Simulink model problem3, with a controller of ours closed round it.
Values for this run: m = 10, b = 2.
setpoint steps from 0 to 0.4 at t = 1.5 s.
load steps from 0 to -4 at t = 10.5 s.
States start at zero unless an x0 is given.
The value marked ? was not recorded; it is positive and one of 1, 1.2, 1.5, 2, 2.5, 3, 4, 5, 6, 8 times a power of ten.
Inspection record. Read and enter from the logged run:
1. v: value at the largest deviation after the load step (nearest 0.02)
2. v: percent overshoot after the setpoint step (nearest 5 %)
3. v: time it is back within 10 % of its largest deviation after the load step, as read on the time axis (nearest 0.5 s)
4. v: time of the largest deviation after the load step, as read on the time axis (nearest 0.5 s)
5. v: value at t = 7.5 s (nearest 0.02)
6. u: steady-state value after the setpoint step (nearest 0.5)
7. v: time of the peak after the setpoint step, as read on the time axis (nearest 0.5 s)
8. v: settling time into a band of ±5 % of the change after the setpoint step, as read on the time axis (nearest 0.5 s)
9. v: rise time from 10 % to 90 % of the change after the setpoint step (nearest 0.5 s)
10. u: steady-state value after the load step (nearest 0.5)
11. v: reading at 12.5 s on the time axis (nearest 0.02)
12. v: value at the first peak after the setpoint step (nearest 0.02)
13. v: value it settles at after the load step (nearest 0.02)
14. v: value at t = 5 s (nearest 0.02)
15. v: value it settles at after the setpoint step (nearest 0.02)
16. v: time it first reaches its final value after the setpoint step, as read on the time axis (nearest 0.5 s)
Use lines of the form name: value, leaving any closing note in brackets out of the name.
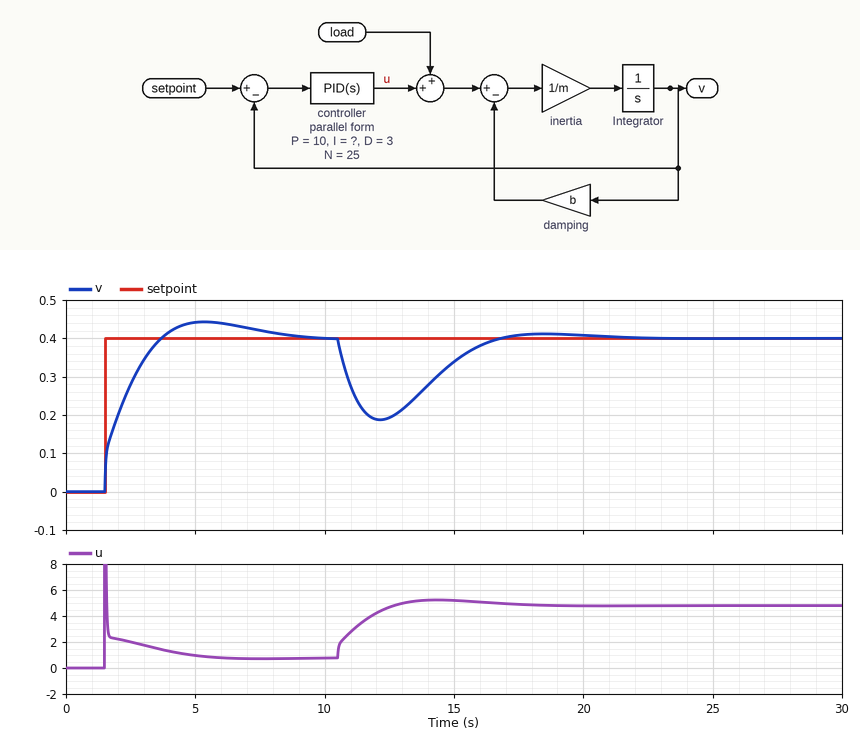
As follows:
v: value at the largest deviation after the load step: 0.18
v: percent overshoot after the setpoint step: 10 %
v: time it is back within 10 % of its largest deviation after the load step, as read on the time axis: 16.0 s
v: time of the largest deviation after the load step, as read on the time axis: 12.0 s
v: value at t = 7.5 s: 0.42
u: steady-state value after the setpoint step: 1.0
v: time of the peak after the setpoint step, as read on the time axis: 5.5 s
v: settling time into a band of ±5 % of the change after the setpoint step, as read on the time axis: 7.5 s
v: rise time from 10 % to 90 % of the change after the setpoint step: 1.5 s
u: steady-state value after the load step: 5.0
v: reading at 12.5 s on the time axis: 0.20
v: value at the first peak after the setpoint step: 0.44
v: value it settles at after the load step: 0.40
v: value at t = 5 s: 0.44
v: value it settles at after the setpoint step: 0.40
v: time it first reaches its final value after the setpoint step, as read on the time axis: 3.5 s
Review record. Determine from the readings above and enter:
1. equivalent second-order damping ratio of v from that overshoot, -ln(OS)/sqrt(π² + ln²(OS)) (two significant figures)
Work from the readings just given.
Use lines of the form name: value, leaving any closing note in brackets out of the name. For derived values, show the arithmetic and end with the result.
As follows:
equivalent second-order damping ratio of v from that overshoot, -ln(OS)/sqrt(π² + ln²(OS)): ln(0.1) = -2.303; 2.303 / sqrt(9.870 + 5.302) = 0.59
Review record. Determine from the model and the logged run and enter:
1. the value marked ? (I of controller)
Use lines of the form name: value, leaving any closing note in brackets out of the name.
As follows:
the value marked ?: 6
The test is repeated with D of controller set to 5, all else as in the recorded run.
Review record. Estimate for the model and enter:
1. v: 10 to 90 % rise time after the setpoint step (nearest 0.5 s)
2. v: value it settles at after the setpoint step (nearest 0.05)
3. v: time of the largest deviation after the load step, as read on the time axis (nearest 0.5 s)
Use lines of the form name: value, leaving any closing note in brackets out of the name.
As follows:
v: 10 to 90 % rise time after the setpoint step: 2.0 s
v: value it settles at after the setpoint step: 0.40
v: time of the largest deviation after the load step, as read on the time axis: 12.5 s
